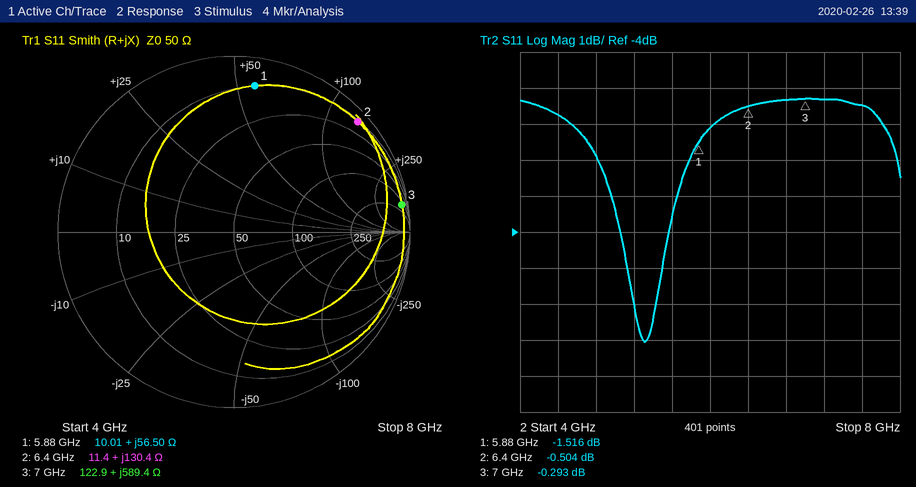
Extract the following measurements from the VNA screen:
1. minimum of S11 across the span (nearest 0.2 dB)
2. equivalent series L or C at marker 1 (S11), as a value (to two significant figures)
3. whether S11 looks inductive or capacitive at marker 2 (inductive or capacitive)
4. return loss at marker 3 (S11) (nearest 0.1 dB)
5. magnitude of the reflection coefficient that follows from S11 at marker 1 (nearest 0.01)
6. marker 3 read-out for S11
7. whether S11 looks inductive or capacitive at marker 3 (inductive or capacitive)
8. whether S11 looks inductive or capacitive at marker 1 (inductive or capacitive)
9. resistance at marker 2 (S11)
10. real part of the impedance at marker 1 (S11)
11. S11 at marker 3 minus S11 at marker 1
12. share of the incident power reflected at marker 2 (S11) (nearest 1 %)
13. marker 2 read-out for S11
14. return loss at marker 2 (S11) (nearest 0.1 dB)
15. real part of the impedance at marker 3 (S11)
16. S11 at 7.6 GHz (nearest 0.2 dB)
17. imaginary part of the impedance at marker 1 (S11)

-7.0 dB
1.5 nH
inductive
0.3 dB
0.84
-0.293 dB
inductive
inductive
11.4 Ω
10.01 Ω
1.223 dB
89 %
-0.504 dB
0.5 dB
122.9 Ω
-0.4 dB
+56.50 Ω
